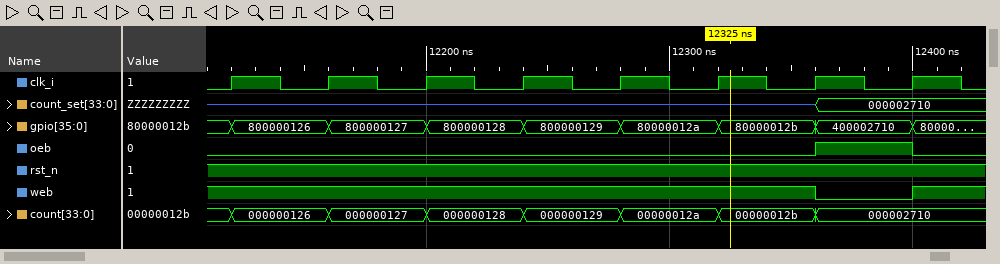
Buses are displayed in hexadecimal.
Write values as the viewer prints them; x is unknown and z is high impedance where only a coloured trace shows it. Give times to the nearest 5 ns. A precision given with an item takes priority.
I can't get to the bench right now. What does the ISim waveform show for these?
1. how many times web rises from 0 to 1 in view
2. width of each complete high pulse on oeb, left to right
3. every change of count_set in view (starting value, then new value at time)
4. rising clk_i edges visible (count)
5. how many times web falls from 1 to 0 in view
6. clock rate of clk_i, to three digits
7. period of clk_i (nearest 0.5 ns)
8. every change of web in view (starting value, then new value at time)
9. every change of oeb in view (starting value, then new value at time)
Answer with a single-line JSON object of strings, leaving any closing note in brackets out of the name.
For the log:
{"how many times web rises from 0 to 1 in view": "1", "width of each complete high pulse on oeb, left to right": "40 ns", "every change of count_set in view": "z, 000002710 at 12360 ns", "rising clk_i edges visible": "8", "how many times web falls from 1 to 0 in view": "1", "clock rate of clk_i, to three digits": "25.0 MHz", "period of clk_i": "40 ns", "every change of web in view": "1, 0 at 12360 ns, 1 at 12400 ns", "every change of oeb in view": "0, 1 at 12360 ns, 0 at 12400 ns"}
